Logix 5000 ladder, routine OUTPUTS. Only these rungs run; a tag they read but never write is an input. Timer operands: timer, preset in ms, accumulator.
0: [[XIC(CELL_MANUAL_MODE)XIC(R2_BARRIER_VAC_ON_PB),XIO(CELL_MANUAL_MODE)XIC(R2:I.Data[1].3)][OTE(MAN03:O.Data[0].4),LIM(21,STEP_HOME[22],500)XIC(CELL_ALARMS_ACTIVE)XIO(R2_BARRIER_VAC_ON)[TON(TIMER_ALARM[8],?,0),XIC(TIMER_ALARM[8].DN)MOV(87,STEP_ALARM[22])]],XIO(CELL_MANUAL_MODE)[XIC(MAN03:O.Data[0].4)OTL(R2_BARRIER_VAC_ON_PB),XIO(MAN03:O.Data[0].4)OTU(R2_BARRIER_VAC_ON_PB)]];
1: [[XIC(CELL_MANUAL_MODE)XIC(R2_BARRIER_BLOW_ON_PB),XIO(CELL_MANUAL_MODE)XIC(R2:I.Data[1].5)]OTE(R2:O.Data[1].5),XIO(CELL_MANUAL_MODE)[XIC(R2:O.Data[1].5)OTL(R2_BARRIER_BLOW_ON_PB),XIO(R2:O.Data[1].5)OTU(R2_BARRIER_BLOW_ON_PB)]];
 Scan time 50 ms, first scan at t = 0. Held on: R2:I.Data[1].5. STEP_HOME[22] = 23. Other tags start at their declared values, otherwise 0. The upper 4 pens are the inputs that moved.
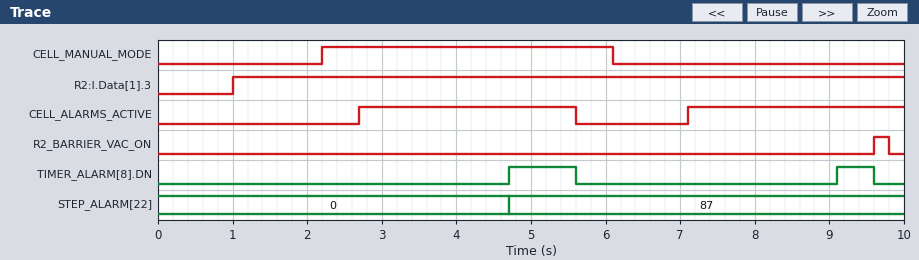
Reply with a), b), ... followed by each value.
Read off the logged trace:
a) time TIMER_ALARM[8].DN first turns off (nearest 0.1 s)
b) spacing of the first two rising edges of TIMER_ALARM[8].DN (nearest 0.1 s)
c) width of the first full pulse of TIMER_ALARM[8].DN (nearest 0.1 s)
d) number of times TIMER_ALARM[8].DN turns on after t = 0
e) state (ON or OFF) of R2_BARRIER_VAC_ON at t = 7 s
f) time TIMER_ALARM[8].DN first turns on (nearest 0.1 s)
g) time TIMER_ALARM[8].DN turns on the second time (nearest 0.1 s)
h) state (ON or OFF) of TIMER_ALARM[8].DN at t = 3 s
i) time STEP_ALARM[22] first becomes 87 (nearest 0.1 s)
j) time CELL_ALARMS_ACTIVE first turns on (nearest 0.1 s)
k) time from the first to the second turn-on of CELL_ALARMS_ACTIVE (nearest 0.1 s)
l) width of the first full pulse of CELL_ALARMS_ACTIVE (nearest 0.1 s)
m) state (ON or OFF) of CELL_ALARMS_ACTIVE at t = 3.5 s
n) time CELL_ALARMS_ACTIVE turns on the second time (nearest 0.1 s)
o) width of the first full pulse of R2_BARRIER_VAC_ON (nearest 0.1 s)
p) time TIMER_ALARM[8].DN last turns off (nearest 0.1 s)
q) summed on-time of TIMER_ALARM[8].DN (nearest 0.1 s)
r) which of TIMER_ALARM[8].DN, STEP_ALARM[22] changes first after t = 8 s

a) 5.6 s
b) 4.4 s
c) 0.9 s
d) 2
e) OFF
f) 4.7 s
g) 9.1 s
h) OFF
i) 4.7 s
j) 2.7 s
k) 4.4 s
l) 2.9 s
m) ON
n) 7.1 s
o) 0.2 s
p) 9.6 s
q) 1.4 s
r) TIMER_ALARM[8].DN
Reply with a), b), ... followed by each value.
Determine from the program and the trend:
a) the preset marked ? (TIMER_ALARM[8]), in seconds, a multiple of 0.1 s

a) 2.0 s
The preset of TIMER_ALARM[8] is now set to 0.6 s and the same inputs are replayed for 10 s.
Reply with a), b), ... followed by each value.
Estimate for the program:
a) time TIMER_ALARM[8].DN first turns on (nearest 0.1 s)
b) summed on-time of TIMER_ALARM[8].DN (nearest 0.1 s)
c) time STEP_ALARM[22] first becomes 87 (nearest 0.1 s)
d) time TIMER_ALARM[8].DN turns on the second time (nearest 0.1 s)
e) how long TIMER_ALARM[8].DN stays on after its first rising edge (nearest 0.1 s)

a) 3.3 s
b) 4.2 s
c) 3.3 s
d) 7.7 s
e) 2.3 s
